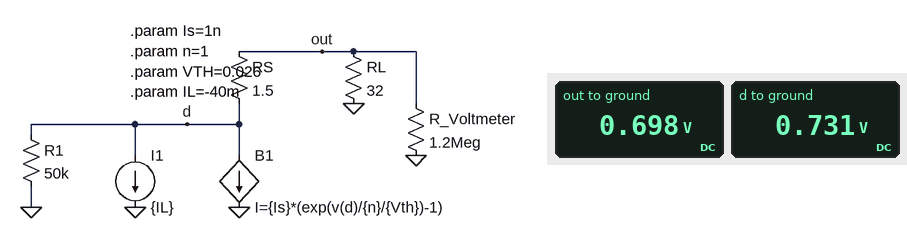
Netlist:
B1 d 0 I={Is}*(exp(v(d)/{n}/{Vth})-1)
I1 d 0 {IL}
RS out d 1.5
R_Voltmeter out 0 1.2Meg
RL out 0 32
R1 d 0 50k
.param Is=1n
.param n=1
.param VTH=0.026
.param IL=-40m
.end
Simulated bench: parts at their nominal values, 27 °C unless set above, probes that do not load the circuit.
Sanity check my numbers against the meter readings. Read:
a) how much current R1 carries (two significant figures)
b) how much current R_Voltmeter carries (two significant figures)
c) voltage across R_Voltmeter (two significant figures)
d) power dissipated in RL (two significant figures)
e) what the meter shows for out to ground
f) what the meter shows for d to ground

15 µA
580 nA
700 mV
15 mW
0.698 V
0.731 V
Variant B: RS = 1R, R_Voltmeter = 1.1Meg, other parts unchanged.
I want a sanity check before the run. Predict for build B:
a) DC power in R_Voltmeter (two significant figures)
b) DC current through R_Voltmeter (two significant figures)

450 nW
640 nA
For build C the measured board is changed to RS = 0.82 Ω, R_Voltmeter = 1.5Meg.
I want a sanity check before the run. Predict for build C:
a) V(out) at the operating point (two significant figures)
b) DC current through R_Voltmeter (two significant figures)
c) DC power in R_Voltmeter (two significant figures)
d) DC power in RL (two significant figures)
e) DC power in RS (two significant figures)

710 mV
470 nA
330 nW
16 mW
400 µW
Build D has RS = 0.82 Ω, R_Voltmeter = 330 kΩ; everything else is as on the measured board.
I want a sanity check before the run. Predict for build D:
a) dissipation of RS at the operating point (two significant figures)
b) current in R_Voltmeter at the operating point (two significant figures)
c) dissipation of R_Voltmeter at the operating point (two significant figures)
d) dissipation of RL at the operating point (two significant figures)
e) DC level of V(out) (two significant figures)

400 µW
2.1 µA
1.5 µW
16 mW
710 mV
